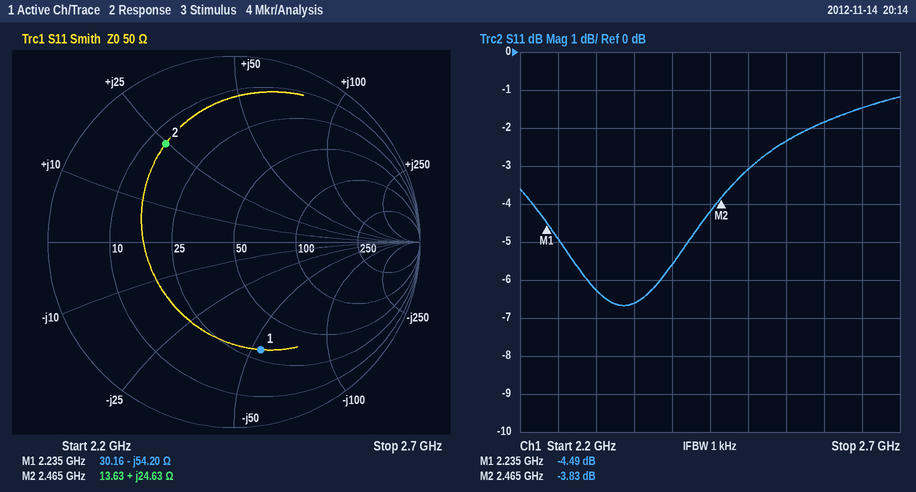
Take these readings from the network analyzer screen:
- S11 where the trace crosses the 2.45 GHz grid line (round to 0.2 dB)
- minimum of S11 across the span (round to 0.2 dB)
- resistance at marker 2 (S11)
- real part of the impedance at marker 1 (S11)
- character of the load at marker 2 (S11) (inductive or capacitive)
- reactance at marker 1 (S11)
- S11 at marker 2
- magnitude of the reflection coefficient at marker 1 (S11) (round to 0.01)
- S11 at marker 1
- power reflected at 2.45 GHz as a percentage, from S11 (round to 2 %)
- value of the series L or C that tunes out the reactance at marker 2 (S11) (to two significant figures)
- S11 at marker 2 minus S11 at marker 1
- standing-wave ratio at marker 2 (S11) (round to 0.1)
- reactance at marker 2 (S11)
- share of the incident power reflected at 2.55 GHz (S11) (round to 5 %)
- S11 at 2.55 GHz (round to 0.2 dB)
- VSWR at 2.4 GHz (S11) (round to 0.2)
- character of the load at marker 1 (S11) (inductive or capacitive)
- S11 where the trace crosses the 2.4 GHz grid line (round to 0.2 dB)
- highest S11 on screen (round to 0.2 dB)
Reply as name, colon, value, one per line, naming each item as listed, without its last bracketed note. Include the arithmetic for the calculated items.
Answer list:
S11 where the trace crosses the 2.45 GHz grid line: -4.2 dB
minimum of S11 across the span: -6.6 dB
resistance at marker 2: 13.63 Ω
real part of the impedance at marker 1: 30.16 Ω
character of the load at marker 2 (S11): inductive
reactance at marker 1: -54.20 Ω
S11 at marker 2: -3.83 dB
magnitude of the reflection coefficient at marker 1 (S11): 0.60
S11 at marker 1: -4.49 dB
power reflected at 2.45 GHz as a percentage, from S11: 10^(-4.2/10) ≈ 38 %
value of the series L or C that tunes out the reactance at marker 2 (S11): C = 1/(2π × 2.465 GHz × 24.63 Ω) ≈ 2.6 pF
S11 at marker 2 minus S11 at marker 1: -3.83 − (-4.49) = 0.66 dB
standing-wave ratio at marker 2 (S11): 4.6
reactance at marker 2: +24.63 Ω
share of the incident power reflected at 2.55 GHz (S11): 10^(-2.4/10) ≈ 57.5 %, so 60 % to the nearest 5 %
S11 at 2.55 GHz: -2.4 dB
VSWR at 2.4 GHz (S11): |Γ| = 10^(-5.6/20) = 0.5248; VSWR = (1 + 0.5248)/(1 − 0.5248) ≈ 3.2
character of the load at marker 1 (S11): capacitive
S11 where the trace crosses the 2.4 GHz grid line: -5.6 dB
highest S11 on screen: -1.2 dB
